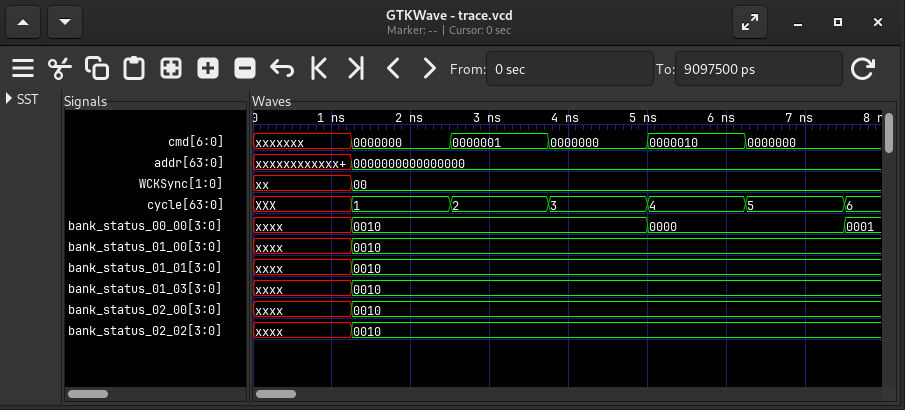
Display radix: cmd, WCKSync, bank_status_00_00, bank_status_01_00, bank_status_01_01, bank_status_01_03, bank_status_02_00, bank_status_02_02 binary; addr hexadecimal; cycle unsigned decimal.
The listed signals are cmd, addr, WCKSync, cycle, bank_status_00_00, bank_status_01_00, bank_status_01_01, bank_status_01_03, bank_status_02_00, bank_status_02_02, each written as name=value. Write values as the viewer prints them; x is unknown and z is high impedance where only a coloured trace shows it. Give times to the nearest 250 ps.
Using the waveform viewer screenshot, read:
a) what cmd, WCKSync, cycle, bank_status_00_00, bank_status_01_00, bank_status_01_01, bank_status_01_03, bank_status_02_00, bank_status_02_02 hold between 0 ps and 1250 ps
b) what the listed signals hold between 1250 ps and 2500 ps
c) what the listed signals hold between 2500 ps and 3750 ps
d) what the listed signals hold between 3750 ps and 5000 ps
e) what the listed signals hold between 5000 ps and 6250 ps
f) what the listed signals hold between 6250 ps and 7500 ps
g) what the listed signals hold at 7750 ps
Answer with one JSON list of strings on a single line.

["cmd=xxxxxxx, WCKSync=xx, cycle=XXX, bank_status_00_00=xxxx, bank_status_01_00=xxxx, bank_status_01_01=xxxx, bank_status_01_03=xxxx, bank_status_02_00=xxxx, bank_status_02_02=xxxx", "cmd=0000000, addr=0000000000000000, WCKSync=00, cycle=1, bank_status_00_00=0010, bank_status_01_00=0010, bank_status_01_01=0010, bank_status_01_03=0010, bank_status_02_00=0010, bank_status_02_02=0010", "cmd=0000001, addr=0000000000000000, WCKSync=00, cycle=2, bank_status_00_00=0010, bank_status_01_00=0010, bank_status_01_01=0010, bank_status_01_03=0010, bank_status_02_00=0010, bank_status_02_02=0010", "cmd=0000000, addr=0000000000000000, WCKSync=00, cycle=3, bank_status_00_00=0010, bank_status_01_00=0010, bank_status_01_01=0010, bank_status_01_03=0010, bank_status_02_00=0010, bank_status_02_02=0010", "cmd=0000010, addr=0000000000000000, WCKSync=00, cycle=4, bank_status_00_00=0000, bank_status_01_00=0010, bank_status_01_01=0010, bank_status_01_03=0010, bank_status_02_00=0010, bank_status_02_02=0010", "cmd=0000000, addr=0000000000000000, WCKSync=00, cycle=5, bank_status_00_00=0000, bank_status_01_00=0010, bank_status_01_01=0010, bank_status_01_03=0010, bank_status_02_00=0010, bank_status_02_02=0010", "cmd=0000000, addr=0000000000000000, WCKSync=00, cycle=6, bank_status_00_00=0001, bank_status_01_00=0010, bank_status_01_01=0010, bank_status_01_03=0010, bank_status_02_00=0010, bank_status_02_02=0010"]
